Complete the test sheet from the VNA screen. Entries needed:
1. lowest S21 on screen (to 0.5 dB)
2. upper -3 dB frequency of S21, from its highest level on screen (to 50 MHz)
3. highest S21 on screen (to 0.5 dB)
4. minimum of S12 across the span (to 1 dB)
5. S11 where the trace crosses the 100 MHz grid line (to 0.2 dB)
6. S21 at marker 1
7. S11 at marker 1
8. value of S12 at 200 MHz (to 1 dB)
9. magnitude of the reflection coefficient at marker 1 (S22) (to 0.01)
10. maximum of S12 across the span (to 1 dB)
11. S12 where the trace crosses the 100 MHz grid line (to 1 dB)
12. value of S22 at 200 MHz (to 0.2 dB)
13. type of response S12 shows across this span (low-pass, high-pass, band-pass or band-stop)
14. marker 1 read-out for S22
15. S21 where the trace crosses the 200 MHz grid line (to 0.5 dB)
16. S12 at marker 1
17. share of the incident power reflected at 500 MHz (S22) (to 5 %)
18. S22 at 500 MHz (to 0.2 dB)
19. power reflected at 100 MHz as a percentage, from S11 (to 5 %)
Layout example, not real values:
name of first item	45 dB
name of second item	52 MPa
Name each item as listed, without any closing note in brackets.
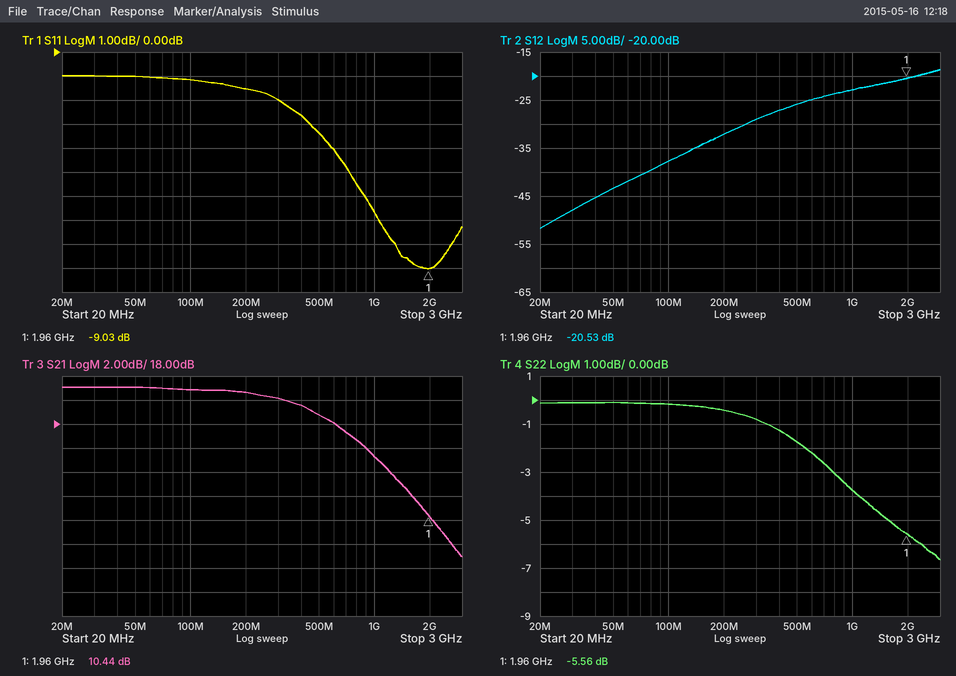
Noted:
lowest S21 on screen	7.0 dB
upper -3 dB frequency of S21, from its highest level on screen	600 MHz
highest S21 on screen	21.0 dB
minimum of S12 across the span	-52 dB
S11 where the trace crosses the 100 MHz grid line	-1.2 dB
S21 at marker 1	10.44 dB
S11 at marker 1	-9.03 dB
value of S12 at 200 MHz	-32 dB
magnitude of the reflection coefficient at marker 1 (S22)	0.53
maximum of S12 across the span	-19 dB
S12 where the trace crosses the 100 MHz grid line	-38 dB
value of S22 at 200 MHz	-0.4 dB
type of response S12 shows across this span	high-pass
marker 1 read-out for S22	-5.56 dB
S21 where the trace crosses the 200 MHz grid line	20.5 dB
S12 at marker 1	-20.53 dB
share of the incident power reflected at 500 MHz (S22)	65 %
S22 at 500 MHz	-1.8 dB
power reflected at 100 MHz as a percentage, from S11	75 %
